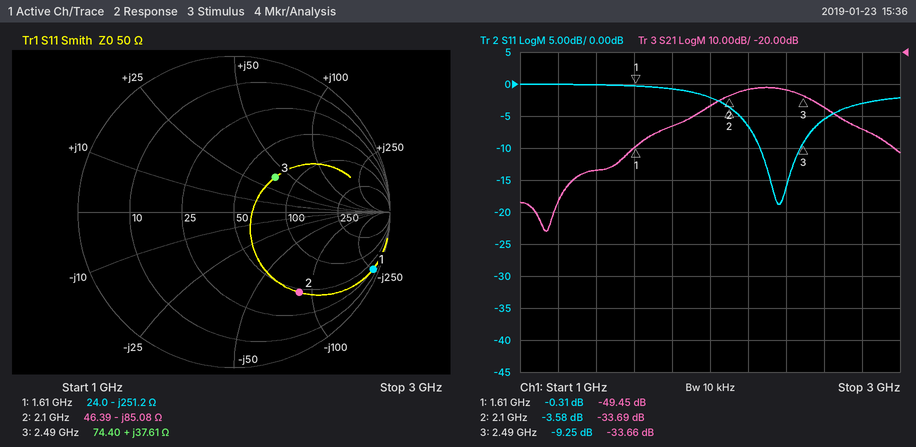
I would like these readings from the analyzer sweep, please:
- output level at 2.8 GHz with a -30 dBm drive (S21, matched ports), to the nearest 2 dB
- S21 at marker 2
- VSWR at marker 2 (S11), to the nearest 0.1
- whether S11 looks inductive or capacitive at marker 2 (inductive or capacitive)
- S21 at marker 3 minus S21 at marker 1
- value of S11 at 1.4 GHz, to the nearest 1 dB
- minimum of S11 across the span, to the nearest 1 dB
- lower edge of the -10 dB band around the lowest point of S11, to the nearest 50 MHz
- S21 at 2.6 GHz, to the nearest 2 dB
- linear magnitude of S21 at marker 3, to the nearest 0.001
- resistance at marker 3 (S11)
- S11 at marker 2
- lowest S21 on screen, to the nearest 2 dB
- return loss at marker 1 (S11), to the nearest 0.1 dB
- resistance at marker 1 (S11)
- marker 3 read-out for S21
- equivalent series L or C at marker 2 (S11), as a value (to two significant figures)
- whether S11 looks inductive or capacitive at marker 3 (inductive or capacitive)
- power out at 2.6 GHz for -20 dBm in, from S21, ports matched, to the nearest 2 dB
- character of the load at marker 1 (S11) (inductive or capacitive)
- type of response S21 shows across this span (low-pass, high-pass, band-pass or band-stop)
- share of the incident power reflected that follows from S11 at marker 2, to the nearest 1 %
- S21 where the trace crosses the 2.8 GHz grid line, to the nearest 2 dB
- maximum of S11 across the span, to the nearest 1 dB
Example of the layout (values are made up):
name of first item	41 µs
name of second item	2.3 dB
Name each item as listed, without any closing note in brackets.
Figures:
output level at 2.8 GHz with a -30 dBm drive (S21, matched ports), to the nearest 2 dB	-74 dBm
S21 at marker 2	-33.69 dB
VSWR at marker 2 (S11), to the nearest 0.1	4.9
whether S11 looks inductive or capacitive at marker 2	capacitive
S21 at marker 3 minus S21 at marker 1	15.79 dB
value of S11 at 1.4 GHz, to the nearest 1 dB	0 dB
minimum of S11 across the span, to the nearest 1 dB	-19 dB
lower edge of the -10 dB band around the lowest point of S11, to the nearest 50 MHz	2.25 GHz
S21 at 2.6 GHz, to the nearest 2 dB	-38 dB
linear magnitude of S21 at marker 3, to the nearest 0.001	0.021
resistance at marker 3	74.40 Ω
S11 at marker 2	-3.58 dB
lowest S21 on screen, to the nearest 2 dB	-76 dB
return loss at marker 1 (S11), to the nearest 0.1 dB	0.3 dB
resistance at marker 1	24.0 Ω
marker 3 read-out for S21	-33.66 dB
equivalent series L or C at marker 2 (S11), as a value	890 fF
whether S11 looks inductive or capacitive at marker 3	inductive
power out at 2.6 GHz for -20 dBm in, from S21, ports matched, to the nearest 2 dB	-58 dBm
character of the load at marker 1 (S11)	capacitive
type of response S21 shows across this span	band-pass
share of the incident power reflected that follows from S11 at marker 2, to the nearest 1 %	44 %
S21 where the trace crosses the 2.8 GHz grid line, to the nearest 2 dB	-44 dB
maximum of S11 across the span, to the nearest 1 dB	0 dB
